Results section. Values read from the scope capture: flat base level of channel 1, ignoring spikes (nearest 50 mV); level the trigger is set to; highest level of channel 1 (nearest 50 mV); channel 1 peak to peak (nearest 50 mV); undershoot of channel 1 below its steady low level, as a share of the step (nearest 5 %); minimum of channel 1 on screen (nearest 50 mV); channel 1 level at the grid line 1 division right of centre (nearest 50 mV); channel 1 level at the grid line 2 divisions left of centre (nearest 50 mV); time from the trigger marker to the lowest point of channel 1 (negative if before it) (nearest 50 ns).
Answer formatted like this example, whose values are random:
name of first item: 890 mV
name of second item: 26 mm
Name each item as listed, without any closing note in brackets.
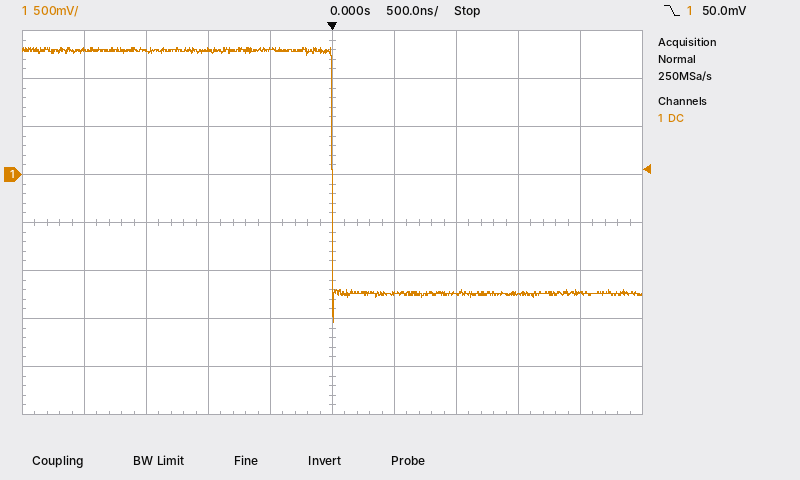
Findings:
flat base level of channel 1, ignoring spikes: -1.25 V
level the trigger is set to: 50.0 mV
highest level of channel 1: 1.30 V
channel 1 peak to peak: 2.85 V
undershoot of channel 1 below its steady low level, as a share of the step: 10 %
minimum of channel 1 on screen: -1.55 V
channel 1 level at the grid line 1 division right of centre: -1.25 V
channel 1 level at the grid line 2 divisions left of centre: 1.30 V
time from the trigger marker to the lowest point of channel 1 (negative if before it): 0 ns
